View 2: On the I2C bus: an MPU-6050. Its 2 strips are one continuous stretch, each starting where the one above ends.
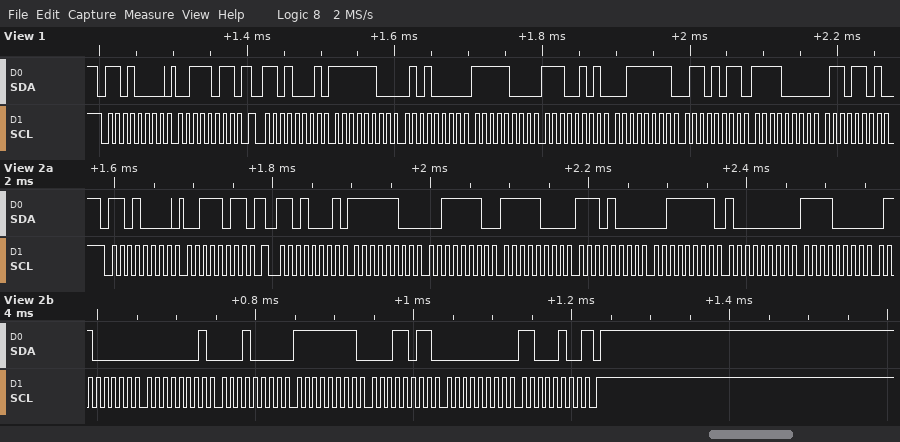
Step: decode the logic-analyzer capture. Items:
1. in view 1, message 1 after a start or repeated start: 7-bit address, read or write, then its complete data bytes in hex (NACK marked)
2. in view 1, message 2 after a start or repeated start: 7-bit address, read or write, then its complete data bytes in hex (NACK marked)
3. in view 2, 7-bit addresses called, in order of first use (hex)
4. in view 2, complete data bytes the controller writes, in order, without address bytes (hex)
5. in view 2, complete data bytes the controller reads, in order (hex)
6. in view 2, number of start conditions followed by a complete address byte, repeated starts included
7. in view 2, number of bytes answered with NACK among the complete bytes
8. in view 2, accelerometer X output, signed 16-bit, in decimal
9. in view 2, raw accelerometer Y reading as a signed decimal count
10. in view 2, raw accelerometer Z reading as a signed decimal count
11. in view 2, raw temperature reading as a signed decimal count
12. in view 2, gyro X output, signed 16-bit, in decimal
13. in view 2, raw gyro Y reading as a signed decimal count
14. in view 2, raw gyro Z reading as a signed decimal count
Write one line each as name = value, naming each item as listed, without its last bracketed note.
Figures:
in view 1, message 1 after a start or repeated start: 7-bit address, read or write, then its complete data bytes in hex = 0x68 write: 3B
in view 1, message 2 after a start or repeated start: 7-bit address, read or write, then its complete data bytes in hex = 0x68 read: FC 50 F8 E5 3F 6B F0 6D
in view 2, 7-bit addresses called, in order of first use = 0x68
in view 2, complete data bytes the controller writes, in order, without address bytes = 3B
in view 2, complete data bytes the controller reads, in order = FC 3E F8 E8 3F 80 F0 60 01 10 FF 1B 00 C4
in view 2, number of start conditions followed by a complete address byte, repeated starts included = 2
in view 2, number of bytes answered with NACK among the complete bytes = 1
in view 2, accelerometer X output, signed 16-bit, in decimal = -962
in view 2, raw accelerometer Y reading as a signed decimal count = -1816
in view 2, raw accelerometer Z reading as a signed decimal count = 16256
in view 2, raw temperature reading as a signed decimal count = -4000
in view 2, gyro X output, signed 16-bit, in decimal = 272
in view 2, raw gyro Y reading as a signed decimal count = -229
in view 2, raw gyro Z reading as a signed decimal count = 196
